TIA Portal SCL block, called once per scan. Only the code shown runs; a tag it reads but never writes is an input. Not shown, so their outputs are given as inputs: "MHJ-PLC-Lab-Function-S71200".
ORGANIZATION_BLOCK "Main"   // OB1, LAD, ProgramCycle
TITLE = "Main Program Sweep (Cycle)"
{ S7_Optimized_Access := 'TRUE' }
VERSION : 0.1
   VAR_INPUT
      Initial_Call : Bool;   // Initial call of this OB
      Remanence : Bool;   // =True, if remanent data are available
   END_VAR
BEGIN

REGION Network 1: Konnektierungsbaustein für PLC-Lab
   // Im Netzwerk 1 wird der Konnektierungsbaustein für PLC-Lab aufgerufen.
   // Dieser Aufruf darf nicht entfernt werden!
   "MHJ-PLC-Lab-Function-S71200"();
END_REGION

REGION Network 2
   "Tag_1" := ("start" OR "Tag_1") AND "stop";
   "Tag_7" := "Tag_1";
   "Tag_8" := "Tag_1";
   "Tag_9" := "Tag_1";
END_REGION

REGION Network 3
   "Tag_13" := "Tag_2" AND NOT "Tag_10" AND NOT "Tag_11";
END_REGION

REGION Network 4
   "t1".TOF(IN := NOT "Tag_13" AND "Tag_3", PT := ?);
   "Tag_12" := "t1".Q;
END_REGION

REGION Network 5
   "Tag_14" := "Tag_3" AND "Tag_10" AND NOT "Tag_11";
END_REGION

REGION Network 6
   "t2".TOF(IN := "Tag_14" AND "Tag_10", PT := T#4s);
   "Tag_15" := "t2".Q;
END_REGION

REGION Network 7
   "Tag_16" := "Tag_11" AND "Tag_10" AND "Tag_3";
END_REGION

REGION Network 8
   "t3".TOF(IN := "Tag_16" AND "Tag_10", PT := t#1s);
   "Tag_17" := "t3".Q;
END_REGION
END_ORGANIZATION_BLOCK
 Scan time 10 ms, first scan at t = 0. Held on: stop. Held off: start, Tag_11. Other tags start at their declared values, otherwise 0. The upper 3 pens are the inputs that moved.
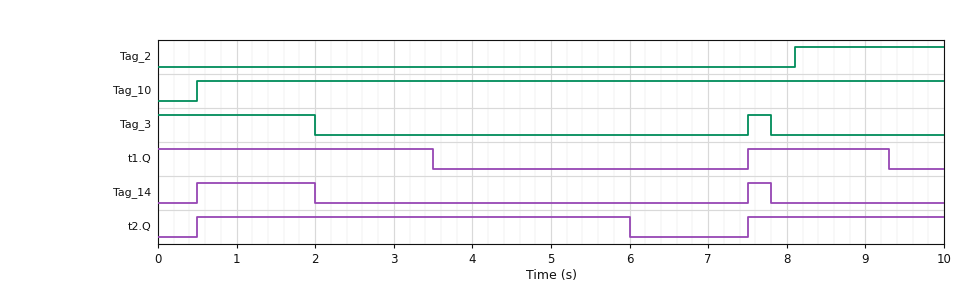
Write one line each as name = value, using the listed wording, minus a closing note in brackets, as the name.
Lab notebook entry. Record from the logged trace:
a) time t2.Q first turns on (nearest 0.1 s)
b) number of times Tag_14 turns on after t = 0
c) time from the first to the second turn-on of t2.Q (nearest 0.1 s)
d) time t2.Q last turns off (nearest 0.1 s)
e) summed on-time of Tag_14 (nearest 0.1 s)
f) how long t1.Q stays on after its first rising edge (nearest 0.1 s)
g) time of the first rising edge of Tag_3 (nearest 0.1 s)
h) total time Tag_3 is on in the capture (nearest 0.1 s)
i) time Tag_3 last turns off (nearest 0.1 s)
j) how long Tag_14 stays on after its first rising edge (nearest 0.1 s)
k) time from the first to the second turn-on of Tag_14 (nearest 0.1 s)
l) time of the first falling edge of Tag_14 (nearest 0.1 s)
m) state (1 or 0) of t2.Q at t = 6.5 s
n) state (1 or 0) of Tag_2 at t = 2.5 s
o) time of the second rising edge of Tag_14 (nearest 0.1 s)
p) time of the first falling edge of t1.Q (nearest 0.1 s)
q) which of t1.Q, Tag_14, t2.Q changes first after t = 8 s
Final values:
time t2.Q first turns on = 0.5 s
number of times Tag_14 turns on after t = 0 = 2
time from the first to the second turn-on of t2.Q = 7.0 s
time t2.Q last turns off = 6.0 s
summed on-time of Tag_14 = 1.8 s
how long t1.Q stays on after its first rising edge = 1.8 s
time of the first rising edge of Tag_3 = 7.5 s
total time Tag_3 is on in the capture = 2.3 s
time Tag_3 last turns off = 7.8 s
how long Tag_14 stays on after its first rising edge = 1.5 s
time from the first to the second turn-on of Tag_14 = 7.0 s
time of the first falling edge of Tag_14 = 2.0 s
state (1 or 0) of t2.Q at t = 6.5 s = 0
state (1 or 0) of Tag_2 at t = 2.5 s = 0
time of the second rising edge of Tag_14 = 7.5 s
time of the first falling edge of t1.Q = 3.5 s
which of t1.Q, Tag_14, t2.Q changes first after t = 8 s = t1.Q
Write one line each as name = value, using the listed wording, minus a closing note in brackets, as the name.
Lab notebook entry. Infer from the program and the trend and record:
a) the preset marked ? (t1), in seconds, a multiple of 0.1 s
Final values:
the preset marked ? (t1), in seconds, a multiple of 0.1 s = 1.5 s
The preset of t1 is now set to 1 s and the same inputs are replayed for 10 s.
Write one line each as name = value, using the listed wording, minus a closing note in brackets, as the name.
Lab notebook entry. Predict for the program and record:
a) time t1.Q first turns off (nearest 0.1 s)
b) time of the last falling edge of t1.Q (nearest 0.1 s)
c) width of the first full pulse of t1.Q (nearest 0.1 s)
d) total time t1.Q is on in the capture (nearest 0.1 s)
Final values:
time t1.Q first turns off = 3.0 s
time of the last falling edge of t1.Q = 8.8 s
width of the first full pulse of t1.Q = 1.3 s
total time t1.Q is on in the capture = 4.3 s
